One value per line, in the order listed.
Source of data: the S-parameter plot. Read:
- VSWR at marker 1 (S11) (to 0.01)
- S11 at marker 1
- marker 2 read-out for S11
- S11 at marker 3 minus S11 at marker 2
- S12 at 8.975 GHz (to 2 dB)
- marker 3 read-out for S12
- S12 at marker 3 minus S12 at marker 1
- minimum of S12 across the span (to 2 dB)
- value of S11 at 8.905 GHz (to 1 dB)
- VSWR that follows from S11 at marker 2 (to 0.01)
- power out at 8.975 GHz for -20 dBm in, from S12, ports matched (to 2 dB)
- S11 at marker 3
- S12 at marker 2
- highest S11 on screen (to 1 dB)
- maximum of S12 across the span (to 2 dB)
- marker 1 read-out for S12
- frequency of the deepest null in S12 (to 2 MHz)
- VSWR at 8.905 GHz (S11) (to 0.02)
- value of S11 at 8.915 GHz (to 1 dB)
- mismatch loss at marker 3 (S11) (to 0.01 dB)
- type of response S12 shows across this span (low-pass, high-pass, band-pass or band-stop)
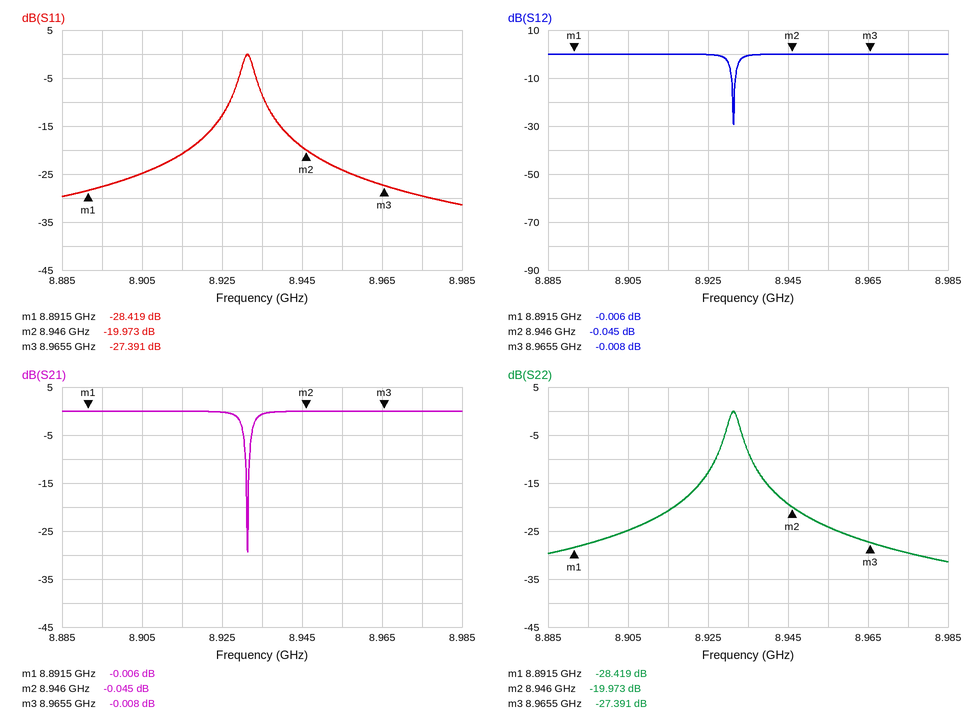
1.08
-28.419 dB
-19.973 dB
-7.418 dB
0 dB
-0.008 dB
-0.002 dB
-30 dB
-25 dB
1.22
-20 dBm
-27.391 dB
-0.045 dB
0 dB
0 dB
-0.006 dB
8.932 GHz
1.12
-21 dB
0.01 dB
band-stop
